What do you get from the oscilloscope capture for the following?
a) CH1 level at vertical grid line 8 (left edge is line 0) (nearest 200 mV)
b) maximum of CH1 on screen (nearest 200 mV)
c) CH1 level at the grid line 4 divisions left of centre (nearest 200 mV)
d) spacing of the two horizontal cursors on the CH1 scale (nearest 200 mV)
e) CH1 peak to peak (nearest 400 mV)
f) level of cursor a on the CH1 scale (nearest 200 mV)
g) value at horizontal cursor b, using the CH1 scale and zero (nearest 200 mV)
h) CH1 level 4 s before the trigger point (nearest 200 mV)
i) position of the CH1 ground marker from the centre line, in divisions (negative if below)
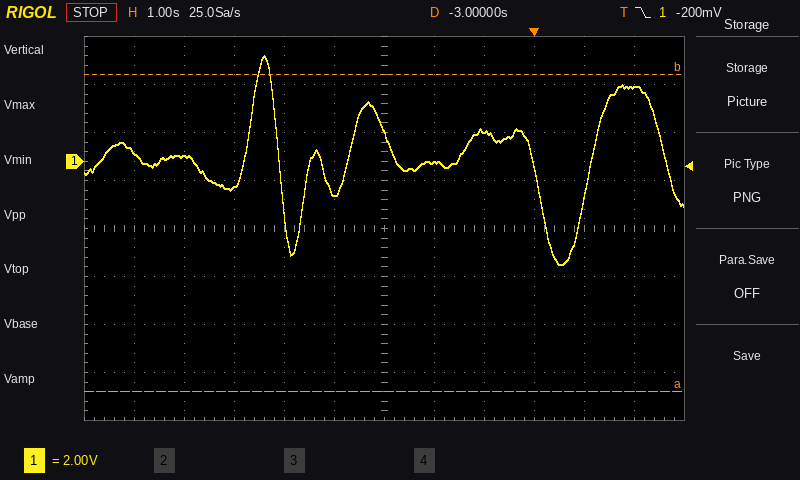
1.2 V
4.4 V
200 mV
13.2 V
8.8 V
-9.6 V
3.6 V
-1.4 V
+1.4 div
